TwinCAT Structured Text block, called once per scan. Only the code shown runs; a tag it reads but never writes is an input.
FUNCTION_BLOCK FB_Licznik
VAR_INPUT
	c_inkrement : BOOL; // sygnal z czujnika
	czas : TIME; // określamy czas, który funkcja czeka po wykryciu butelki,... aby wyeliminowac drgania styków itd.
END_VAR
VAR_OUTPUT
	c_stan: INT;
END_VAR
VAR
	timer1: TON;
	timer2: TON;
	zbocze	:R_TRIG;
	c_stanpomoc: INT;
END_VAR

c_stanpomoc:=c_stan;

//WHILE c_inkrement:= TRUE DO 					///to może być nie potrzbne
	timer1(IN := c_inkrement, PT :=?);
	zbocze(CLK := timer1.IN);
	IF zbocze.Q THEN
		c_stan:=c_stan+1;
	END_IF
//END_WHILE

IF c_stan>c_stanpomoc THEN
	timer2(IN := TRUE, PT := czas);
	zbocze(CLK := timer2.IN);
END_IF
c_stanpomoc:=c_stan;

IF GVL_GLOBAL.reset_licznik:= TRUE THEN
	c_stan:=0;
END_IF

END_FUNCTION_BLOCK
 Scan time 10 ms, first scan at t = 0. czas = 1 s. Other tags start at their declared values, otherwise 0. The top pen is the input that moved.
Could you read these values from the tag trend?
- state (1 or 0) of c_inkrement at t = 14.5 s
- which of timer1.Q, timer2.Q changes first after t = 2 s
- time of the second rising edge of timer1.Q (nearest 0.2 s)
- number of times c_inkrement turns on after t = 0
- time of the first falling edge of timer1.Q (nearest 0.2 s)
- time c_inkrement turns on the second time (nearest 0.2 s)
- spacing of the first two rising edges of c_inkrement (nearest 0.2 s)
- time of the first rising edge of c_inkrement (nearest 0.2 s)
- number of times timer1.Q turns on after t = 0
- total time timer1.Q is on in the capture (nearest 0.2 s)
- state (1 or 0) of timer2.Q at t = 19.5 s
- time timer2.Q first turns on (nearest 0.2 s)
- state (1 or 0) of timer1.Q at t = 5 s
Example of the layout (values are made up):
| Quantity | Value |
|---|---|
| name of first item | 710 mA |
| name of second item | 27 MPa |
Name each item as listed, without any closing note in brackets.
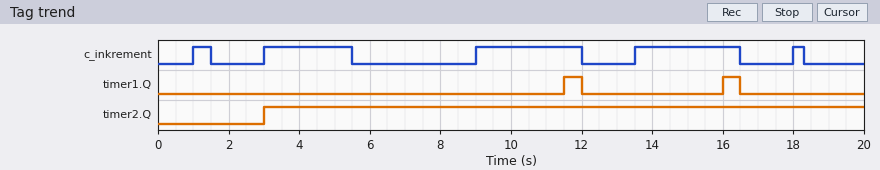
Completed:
| Quantity | Value |
|---|---|
| state (1 or 0) of c_inkrement at t = 14.5 s | 1 |
| which of timer1.Q, timer2.Q changes first after t = 2 s | timer2.Q |
| time of the second rising edge of timer1.Q | 16.0 s |
| number of times c_inkrement turns on after t = 0 | 5 |
| time of the first falling edge of timer1.Q | 12.0 s |
| time c_inkrement turns on the second time | 3.0 s |
| spacing of the first two rising edges of c_inkrement | 2.0 s |
| time of the first rising edge of c_inkrement | 1.0 s |
| number of times timer1.Q turns on after t = 0 | 2 |
| total time timer1.Q is on in the capture | 1.0 s |
| state (1 or 0) of timer2.Q at t = 19.5 s | 1 |
| time timer2.Q first turns on | 3.0 s |
| state (1 or 0) of timer1.Q at t = 5 s | 0 |
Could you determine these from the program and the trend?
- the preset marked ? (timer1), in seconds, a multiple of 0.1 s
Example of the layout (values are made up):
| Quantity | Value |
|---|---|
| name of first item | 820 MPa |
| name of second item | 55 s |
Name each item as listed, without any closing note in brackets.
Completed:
| Quantity | Value |
|---|---|
| the preset marked ? (timer1), in seconds, a multiple of 0.1 s | 2.5 s |
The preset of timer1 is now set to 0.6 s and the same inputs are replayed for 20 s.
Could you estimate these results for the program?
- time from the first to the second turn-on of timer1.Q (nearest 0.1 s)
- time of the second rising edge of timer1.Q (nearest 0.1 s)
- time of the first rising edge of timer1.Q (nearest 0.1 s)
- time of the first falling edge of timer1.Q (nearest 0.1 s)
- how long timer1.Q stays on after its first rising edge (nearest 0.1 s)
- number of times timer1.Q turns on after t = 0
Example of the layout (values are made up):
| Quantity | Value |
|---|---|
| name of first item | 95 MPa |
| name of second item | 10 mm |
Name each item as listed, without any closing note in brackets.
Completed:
| Quantity | Value |
|---|---|
| time from the first to the second turn-on of timer1.Q | 6.0 s |
| time of the second rising edge of timer1.Q | 9.6 s |
| time of the first rising edge of timer1.Q | 3.6 s |
| time of the first falling edge of timer1.Q | 5.5 s |
| how long timer1.Q stays on after its first rising edge | 1.9 s |
| number of times timer1.Q turns on after t = 0 | 3 |
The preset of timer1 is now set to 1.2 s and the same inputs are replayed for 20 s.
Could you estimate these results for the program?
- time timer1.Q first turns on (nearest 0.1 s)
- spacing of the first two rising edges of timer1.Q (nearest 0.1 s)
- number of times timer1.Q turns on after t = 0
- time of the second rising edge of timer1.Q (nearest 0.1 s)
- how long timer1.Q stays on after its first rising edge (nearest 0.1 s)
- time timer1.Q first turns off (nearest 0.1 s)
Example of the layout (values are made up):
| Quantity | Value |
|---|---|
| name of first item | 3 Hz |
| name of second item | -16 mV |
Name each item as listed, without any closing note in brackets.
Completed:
| Quantity | Value |
|---|---|
| time timer1.Q first turns on | 4.2 s |
| spacing of the first two rising edges of timer1.Q | 6.0 s |
| number of times timer1.Q turns on after t = 0 | 3 |
| time of the second rising edge of timer1.Q | 10.2 s |
| how long timer1.Q stays on after its first rising edge | 1.3 s |
| time timer1.Q first turns off | 5.5 s |
